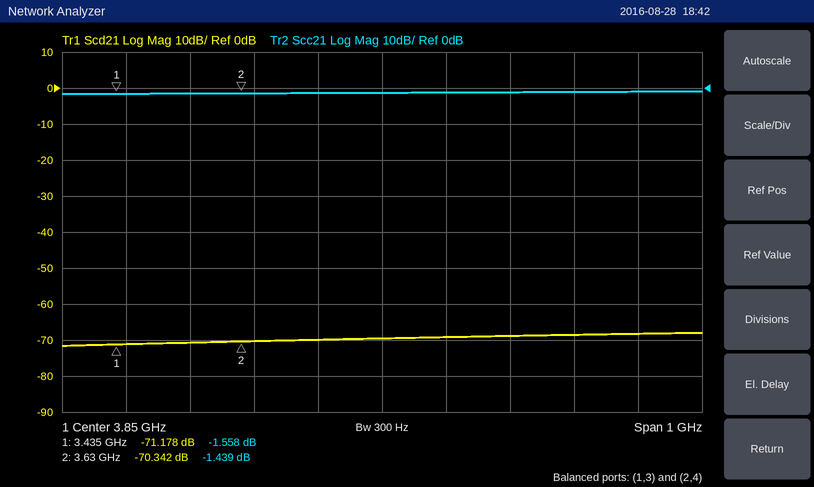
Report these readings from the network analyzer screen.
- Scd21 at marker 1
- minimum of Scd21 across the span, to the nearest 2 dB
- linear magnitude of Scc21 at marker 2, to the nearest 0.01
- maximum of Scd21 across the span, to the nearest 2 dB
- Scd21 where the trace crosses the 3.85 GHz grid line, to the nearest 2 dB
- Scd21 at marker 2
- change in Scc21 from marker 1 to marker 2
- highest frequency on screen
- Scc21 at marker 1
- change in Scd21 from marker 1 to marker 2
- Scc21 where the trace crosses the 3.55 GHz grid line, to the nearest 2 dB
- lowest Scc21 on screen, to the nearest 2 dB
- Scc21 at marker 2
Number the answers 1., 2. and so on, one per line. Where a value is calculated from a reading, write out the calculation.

1. -71.178 dB
2. -72 dB
3. 10^(-1.439/20) ≈ 0.85
4. -68 dB
5. -70 dB
6. -70.342 dB
7. -1.439 − (-1.558) = 0.119 dB
8. 4.35 GHz
9. -1.558 dB
10. -70.342 − (-71.178) = 0.836 dB
11. -2 dB
12. -2 dB
13. -1.439 dB
